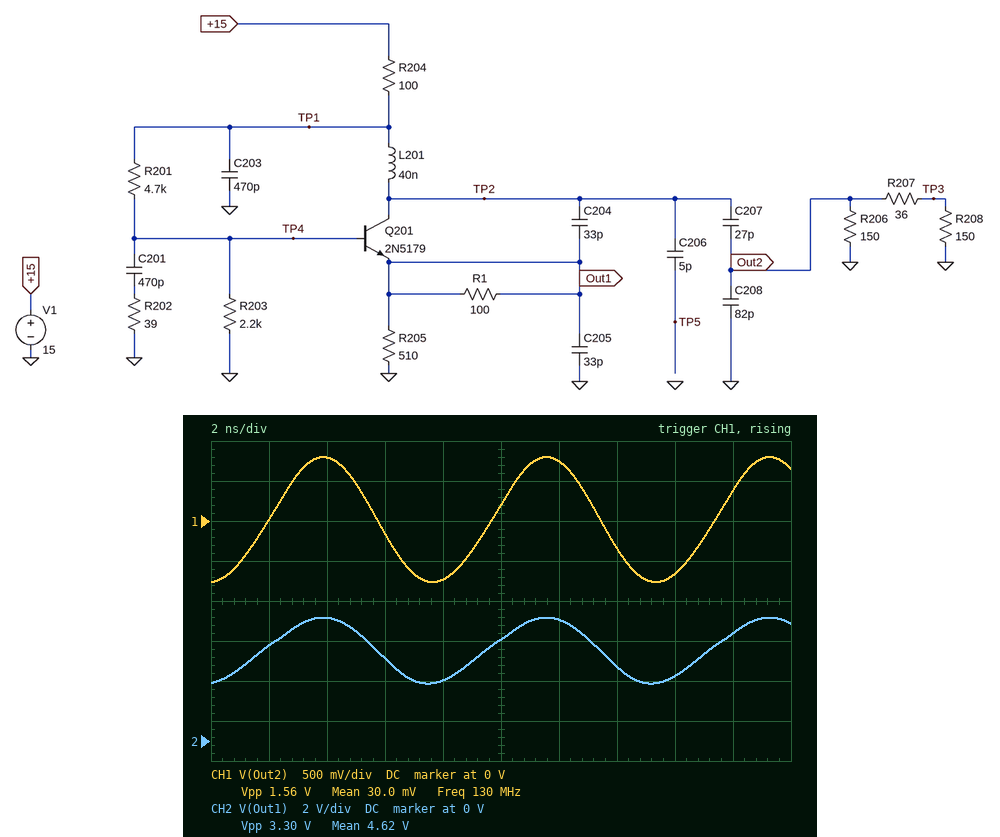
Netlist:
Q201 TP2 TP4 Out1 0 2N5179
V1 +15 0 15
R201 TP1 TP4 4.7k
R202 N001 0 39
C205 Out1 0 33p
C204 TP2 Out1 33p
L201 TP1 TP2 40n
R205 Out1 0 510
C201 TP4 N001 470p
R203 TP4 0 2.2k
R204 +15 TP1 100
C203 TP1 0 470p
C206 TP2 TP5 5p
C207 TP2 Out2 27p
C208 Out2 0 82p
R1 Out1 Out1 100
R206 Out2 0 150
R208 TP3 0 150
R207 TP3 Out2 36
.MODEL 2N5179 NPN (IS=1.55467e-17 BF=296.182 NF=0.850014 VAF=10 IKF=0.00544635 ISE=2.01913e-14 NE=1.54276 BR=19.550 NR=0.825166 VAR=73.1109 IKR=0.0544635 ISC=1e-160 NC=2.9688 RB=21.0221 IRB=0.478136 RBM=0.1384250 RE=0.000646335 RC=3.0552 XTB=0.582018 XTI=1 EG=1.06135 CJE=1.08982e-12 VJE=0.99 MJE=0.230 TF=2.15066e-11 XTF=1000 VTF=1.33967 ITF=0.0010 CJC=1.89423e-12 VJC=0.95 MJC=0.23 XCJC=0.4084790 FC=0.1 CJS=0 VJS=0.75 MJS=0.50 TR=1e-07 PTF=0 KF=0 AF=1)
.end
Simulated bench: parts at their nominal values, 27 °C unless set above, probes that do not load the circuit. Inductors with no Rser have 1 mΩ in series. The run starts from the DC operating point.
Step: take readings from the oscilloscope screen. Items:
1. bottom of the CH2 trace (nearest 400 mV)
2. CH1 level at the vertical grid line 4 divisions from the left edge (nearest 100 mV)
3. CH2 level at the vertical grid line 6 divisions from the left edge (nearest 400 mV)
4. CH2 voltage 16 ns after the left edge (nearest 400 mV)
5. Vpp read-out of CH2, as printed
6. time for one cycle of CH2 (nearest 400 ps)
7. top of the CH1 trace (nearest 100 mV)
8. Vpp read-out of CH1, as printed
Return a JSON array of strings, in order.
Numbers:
["2.8 V", "-700 mV", "6.0 V", "3.2 V", "3.30 V", "7.6 ns", "800 mV", "1.56 V"]
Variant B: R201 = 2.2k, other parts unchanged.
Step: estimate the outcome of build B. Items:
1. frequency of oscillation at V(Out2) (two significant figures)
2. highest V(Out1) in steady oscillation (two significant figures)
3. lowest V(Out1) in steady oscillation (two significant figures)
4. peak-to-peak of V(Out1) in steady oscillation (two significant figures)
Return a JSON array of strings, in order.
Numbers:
["120 MHz", "6.6 V", "5.3 V", "1.3 V"]
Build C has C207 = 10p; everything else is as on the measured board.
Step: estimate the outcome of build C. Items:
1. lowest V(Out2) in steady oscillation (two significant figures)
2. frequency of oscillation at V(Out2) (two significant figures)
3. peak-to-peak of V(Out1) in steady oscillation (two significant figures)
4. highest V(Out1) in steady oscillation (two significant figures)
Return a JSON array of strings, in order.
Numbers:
["-390 mV", "150 MHz", "3.8 V", "6.5 V"]
